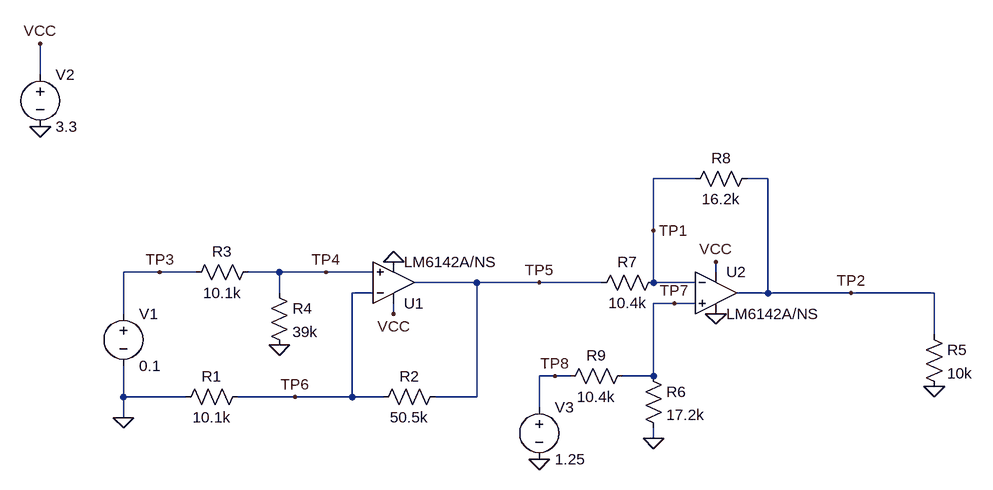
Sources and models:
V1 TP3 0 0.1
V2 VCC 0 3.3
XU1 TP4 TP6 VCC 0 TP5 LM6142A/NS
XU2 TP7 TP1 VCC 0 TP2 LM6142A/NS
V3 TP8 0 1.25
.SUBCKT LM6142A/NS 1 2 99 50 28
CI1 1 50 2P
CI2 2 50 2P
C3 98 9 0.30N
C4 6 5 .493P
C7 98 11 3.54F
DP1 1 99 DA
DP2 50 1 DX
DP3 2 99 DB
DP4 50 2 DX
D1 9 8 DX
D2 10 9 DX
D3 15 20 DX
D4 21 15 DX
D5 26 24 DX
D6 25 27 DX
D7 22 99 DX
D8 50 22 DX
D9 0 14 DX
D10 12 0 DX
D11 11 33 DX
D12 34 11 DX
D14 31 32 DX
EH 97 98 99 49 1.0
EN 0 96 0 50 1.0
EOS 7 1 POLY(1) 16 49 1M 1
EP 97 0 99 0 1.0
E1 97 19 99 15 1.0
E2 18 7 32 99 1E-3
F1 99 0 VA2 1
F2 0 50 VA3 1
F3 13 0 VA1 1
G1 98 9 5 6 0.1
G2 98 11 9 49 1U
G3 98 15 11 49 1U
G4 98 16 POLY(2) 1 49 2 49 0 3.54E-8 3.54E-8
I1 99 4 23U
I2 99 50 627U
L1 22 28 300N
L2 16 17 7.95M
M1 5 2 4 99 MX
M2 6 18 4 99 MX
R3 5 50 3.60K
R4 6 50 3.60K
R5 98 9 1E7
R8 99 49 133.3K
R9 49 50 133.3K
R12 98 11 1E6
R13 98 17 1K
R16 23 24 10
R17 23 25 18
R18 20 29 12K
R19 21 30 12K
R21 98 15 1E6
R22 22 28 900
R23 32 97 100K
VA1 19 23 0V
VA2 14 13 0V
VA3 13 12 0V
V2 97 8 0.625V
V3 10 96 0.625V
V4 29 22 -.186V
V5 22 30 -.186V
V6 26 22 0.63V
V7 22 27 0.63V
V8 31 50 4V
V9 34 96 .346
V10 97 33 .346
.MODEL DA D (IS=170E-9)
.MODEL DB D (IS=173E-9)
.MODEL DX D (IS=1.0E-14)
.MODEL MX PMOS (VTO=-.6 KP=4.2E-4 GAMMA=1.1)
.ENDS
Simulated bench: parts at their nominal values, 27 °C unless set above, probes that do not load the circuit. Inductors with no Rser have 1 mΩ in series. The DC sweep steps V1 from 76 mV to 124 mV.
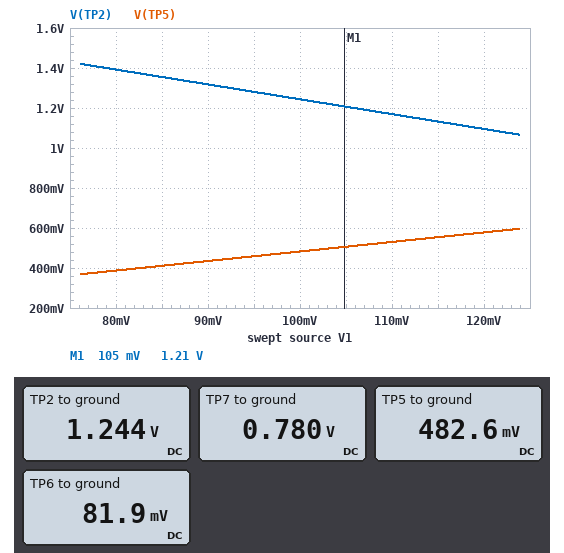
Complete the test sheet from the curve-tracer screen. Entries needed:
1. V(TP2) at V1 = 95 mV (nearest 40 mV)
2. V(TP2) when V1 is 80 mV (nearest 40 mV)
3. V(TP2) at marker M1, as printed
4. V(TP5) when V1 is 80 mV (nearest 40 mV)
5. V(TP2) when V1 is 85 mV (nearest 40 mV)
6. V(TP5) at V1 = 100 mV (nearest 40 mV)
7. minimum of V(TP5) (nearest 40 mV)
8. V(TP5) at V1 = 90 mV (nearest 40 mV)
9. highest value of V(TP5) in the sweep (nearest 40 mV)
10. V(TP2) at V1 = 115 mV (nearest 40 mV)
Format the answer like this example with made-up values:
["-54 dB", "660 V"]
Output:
["1.28 V", "1.40 V", "1.21 V", "400 mV", "1.36 V", "480 mV", "360 mV", "440 mV", "600 mV", "1.12 V"]
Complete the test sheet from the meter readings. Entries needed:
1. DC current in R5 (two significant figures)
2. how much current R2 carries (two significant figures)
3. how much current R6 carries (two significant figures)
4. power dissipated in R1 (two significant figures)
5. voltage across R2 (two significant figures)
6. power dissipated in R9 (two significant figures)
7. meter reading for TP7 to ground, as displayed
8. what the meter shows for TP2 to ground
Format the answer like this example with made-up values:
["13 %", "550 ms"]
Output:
["120 µA", "7.9 µA", "45 µA", "660 nW", "400 mV", "21 µW", "0.780 V", "1.244 V"]
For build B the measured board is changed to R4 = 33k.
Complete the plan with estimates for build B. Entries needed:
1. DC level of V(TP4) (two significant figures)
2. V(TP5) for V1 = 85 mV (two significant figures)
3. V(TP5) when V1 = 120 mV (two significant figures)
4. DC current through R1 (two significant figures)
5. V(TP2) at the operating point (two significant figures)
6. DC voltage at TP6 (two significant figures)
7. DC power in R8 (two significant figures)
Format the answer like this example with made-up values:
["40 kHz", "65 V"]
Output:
["78 mV", "400 mV", "560 mV", "7.8 µA", "1.3 V", "79 mV", "15 µW"]
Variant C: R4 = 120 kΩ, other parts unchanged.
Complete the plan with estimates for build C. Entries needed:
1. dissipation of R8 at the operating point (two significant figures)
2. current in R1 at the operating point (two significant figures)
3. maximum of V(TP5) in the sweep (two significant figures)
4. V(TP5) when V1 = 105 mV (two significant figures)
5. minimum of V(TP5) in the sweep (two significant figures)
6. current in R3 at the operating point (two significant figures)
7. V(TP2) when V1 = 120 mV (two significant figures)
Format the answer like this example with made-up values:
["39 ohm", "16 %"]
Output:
["7.2 µW", "9.4 µA", "690 mV", "590 mV", "430 mV", "610 nA", "950 mV"]
